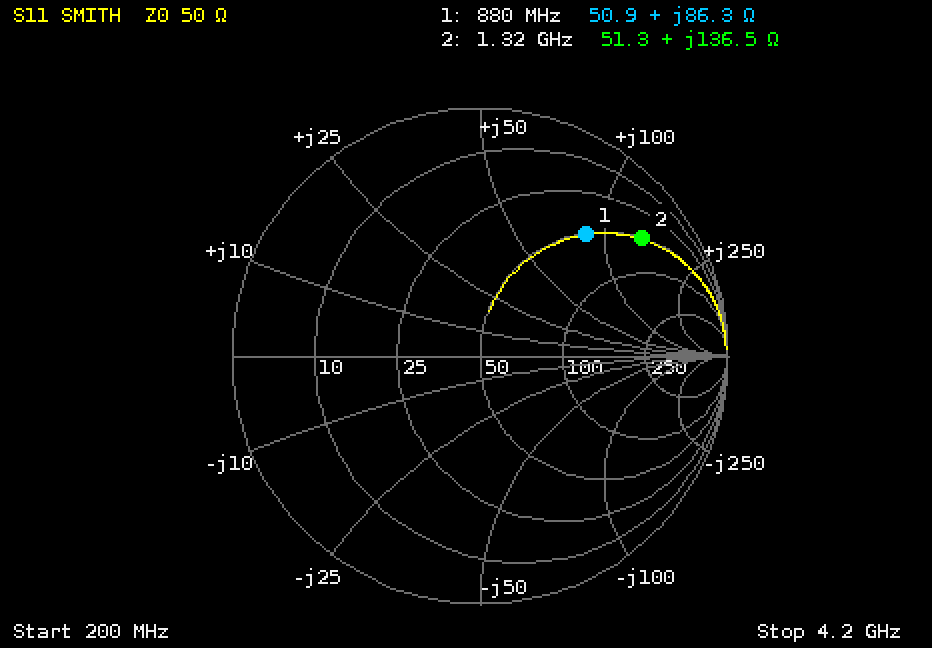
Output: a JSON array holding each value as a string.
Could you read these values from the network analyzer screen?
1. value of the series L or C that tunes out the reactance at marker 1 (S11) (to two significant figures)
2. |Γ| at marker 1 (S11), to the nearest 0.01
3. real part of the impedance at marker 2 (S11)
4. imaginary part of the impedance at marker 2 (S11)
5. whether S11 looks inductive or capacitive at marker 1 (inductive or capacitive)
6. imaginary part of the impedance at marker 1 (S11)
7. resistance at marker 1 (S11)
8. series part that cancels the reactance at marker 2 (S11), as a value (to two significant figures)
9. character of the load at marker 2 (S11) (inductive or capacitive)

["2.1 pF", "0.65", "51.3 Ω", "+136.5 Ω", "inductive", "+86.3 Ω", "50.9 Ω", "880 fF", "inductive"]
